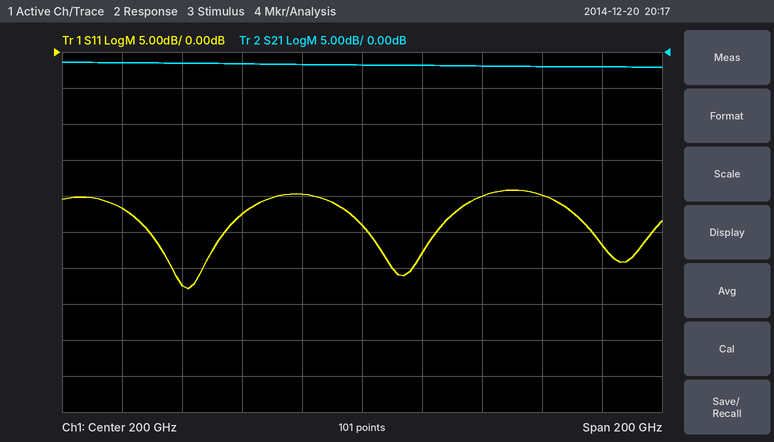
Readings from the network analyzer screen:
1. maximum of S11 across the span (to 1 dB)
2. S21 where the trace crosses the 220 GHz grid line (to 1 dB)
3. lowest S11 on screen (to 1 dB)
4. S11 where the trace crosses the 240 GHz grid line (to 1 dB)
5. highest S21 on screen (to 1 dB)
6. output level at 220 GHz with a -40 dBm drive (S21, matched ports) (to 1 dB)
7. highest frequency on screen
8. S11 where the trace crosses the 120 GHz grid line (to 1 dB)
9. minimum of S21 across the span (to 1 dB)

-19 dB
-2 dB
-33 dB
-20 dB
-1 dB
-42 dBm
300 GHz
-22 dB
-2 dB
